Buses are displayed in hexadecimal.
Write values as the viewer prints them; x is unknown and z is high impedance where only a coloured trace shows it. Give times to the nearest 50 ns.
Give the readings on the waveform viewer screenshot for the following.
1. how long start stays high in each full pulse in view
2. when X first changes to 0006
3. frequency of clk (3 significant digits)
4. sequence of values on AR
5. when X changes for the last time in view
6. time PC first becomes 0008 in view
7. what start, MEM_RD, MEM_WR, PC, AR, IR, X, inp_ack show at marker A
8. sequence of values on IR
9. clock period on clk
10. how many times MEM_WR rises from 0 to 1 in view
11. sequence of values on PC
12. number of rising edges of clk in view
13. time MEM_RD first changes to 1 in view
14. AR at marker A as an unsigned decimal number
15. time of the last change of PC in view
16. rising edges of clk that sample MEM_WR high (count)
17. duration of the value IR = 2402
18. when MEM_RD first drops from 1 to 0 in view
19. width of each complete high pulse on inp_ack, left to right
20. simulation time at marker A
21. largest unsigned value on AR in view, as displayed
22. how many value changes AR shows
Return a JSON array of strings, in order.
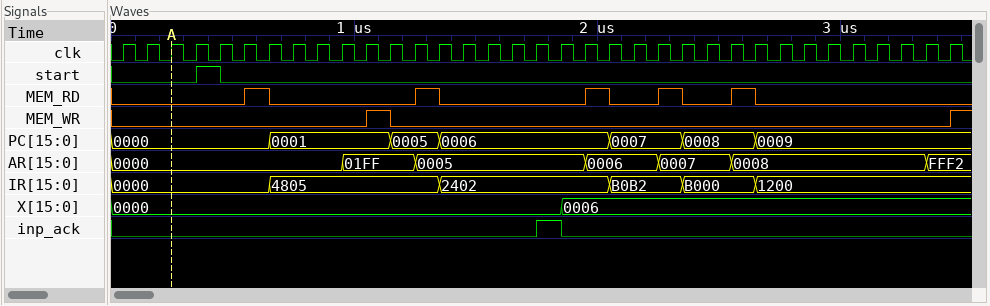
["100 ns", "1850 ns", "10.0 MHz", "0000, 01FF, 0005, 0006, 0007, 0008, FFF2", "1850 ns", "2350 ns", "start=0, MEM_RD=0, MEM_WR=0, PC=0000, AR=0000, IR=0000, X=0000, inp_ack=0", "0000, 4805, 2402, B0B2, B000, 1200", "100 ns", "2", "0000, 0001, 0005, 0006, 0007, 0008, 0009", "35", "550 ns", "0", "2650 ns", "1", "700 ns", "650 ns", "100 ns", "250 ns", "FFF2", "6"]
